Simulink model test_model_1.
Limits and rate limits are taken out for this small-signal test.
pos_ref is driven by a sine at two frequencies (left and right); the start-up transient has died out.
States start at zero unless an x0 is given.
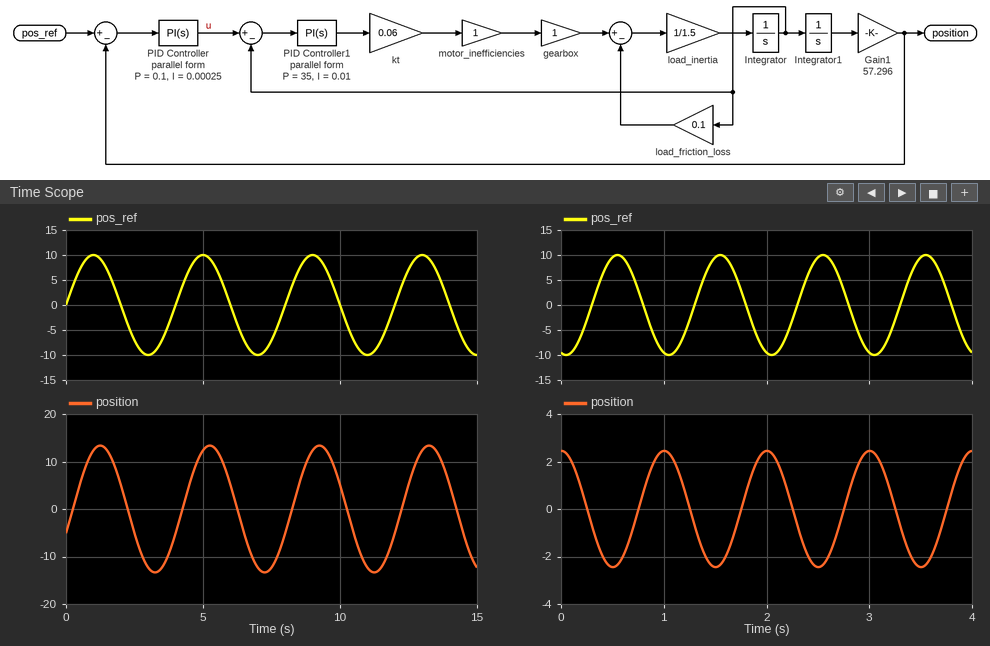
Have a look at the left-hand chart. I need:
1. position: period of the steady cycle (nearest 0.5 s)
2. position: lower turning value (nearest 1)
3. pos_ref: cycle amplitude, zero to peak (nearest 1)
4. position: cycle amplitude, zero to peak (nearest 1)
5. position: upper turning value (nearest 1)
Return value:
4.0 s
-13
10
13
13
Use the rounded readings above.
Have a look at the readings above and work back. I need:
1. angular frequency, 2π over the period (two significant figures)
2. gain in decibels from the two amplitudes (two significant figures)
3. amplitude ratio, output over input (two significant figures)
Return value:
1.6 rad/s
2.3 dB
1.3
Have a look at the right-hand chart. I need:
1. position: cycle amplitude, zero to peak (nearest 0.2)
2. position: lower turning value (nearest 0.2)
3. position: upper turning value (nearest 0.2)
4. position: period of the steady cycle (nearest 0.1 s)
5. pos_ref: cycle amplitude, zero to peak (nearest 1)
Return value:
2.4
-2.4
2.4
1.0 s
10
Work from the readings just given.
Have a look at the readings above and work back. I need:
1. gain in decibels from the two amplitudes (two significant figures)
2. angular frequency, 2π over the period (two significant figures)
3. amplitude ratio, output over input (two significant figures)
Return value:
-12 dB
6.3 rad/s
0.24
